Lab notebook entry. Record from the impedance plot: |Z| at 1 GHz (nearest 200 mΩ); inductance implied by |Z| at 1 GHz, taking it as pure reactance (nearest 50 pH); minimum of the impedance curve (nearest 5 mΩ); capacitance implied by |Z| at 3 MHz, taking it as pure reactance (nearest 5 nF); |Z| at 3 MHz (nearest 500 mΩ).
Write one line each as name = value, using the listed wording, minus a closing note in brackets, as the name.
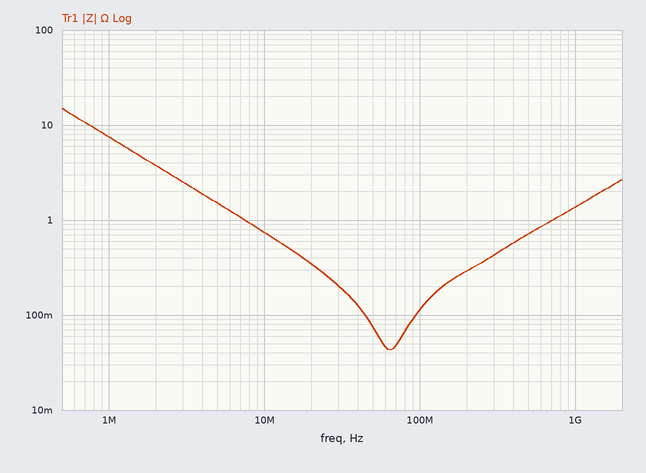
|Z| at 1 GHz = 1.4 Ω
inductance implied by |Z| at 1 GHz, taking it as pure reactance = 200 pH
minimum of the impedance curve = 45 mΩ
capacitance implied by |Z| at 3 MHz, taking it as pure reactance = 20 nF
|Z| at 3 MHz = 2.5 Ω
